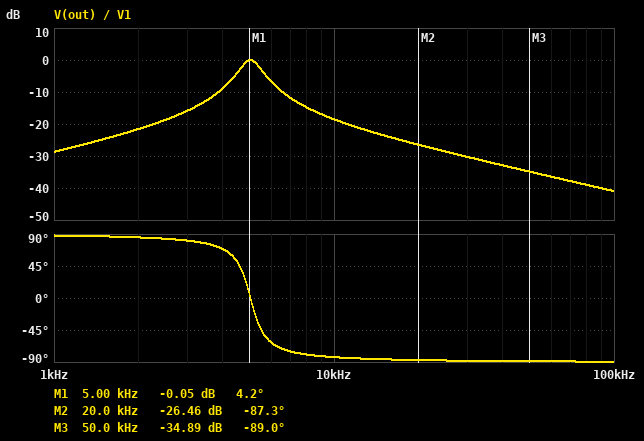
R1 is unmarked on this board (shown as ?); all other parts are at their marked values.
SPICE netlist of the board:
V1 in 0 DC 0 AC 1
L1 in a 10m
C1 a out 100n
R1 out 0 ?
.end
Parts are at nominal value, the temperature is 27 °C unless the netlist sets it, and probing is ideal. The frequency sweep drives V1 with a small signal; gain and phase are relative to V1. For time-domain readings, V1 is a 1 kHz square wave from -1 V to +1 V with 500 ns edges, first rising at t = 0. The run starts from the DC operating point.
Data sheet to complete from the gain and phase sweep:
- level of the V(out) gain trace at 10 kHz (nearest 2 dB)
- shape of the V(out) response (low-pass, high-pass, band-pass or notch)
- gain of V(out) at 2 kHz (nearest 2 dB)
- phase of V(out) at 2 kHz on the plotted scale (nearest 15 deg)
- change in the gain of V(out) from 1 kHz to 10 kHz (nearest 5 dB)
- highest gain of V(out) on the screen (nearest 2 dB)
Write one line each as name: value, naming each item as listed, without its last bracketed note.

level of the V(out) gain trace at 10 kHz: -18 dB
shape of the V(out) response: band-pass
gain of V(out) at 2 kHz: -22 dB
phase of V(out) at 2 kHz on the plotted scale: 90 deg
change in the gain of V(out) from 1 kHz to 10 kHz: 10 dB
highest gain of V(out) on the screen: 0 dB
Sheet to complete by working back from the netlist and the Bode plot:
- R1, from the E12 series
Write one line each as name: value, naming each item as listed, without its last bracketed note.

R1, from the E12 series: 56 Ω
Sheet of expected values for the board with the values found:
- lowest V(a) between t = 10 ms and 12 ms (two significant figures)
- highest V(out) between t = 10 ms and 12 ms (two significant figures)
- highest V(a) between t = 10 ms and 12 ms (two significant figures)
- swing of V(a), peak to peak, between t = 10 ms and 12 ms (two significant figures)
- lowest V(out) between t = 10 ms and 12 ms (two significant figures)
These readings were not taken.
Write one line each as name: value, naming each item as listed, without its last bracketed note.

lowest V(a) between t = 10 ms and 12 ms: -3.0 V
highest V(out) between t = 10 ms and 12 ms: 410 mV
highest V(a) between t = 10 ms and 12 ms: 3.0 V
swing of V(a), peak to peak, between t = 10 ms and 12 ms: 6.1 V
lowest V(out) between t = 10 ms and 12 ms: -410 mV
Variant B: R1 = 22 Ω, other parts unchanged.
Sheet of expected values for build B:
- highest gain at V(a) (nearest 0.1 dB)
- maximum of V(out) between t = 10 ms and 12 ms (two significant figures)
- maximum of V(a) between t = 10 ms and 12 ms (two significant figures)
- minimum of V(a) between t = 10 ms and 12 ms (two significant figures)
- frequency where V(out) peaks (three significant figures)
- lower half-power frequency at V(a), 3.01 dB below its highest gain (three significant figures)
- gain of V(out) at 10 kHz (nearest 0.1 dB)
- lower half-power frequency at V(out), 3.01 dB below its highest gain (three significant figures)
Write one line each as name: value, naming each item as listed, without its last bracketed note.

highest gain at V(a): 23.2 dB
maximum of V(out) between t = 10 ms and 12 ms: 310 mV
maximum of V(a) between t = 10 ms and 12 ms: 5.2 V
minimum of V(a) between t = 10 ms and 12 ms: -5.2 V
frequency where V(out) peaks: 5.03 kHz
lower half-power frequency at V(a), 3.01 dB below its highest gain: 4.85 kHz
gain of V(out) at 10 kHz: -26.6 dB
lower half-power frequency at V(out), 3.01 dB below its highest gain: 4.86 kHz
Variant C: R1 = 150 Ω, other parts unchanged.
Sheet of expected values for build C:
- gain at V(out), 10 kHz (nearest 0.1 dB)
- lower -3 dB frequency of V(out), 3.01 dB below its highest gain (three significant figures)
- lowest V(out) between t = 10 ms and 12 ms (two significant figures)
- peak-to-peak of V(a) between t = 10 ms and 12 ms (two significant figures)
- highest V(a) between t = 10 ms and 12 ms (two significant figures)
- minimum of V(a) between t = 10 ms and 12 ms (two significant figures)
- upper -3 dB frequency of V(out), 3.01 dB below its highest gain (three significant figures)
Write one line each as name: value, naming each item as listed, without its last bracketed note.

gain at V(out), 10 kHz: -10.3 dB
lower -3 dB frequency of V(out), 3.01 dB below its highest gain: 3.98 kHz
lowest V(out) between t = 10 ms and 12 ms: -700 mV
peak-to-peak of V(a) between t = 10 ms and 12 ms: 4.1 V
highest V(a) between t = 10 ms and 12 ms: 2.1 V
minimum of V(a) between t = 10 ms and 12 ms: -2.1 V
upper -3 dB frequency of V(out), 3.01 dB below its highest gain: 6.37 kHz
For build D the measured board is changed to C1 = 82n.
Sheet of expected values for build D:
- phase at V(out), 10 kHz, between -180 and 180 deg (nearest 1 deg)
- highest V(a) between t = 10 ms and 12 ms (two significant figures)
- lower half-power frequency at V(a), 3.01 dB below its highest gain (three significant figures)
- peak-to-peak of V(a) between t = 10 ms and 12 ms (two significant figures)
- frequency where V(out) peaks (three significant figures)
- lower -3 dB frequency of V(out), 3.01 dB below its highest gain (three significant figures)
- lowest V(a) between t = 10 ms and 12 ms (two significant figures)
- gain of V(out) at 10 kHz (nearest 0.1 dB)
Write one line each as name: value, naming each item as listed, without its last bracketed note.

phase at V(out), 10 kHz, between -180 and 180 deg: -83 deg
highest V(a) between t = 10 ms and 12 ms: 2.5 V
lower half-power frequency at V(a), 3.01 dB below its highest gain: 5.06 kHz
peak-to-peak of V(a) between t = 10 ms and 12 ms: 5.0 V
frequency where V(out) peaks: 5.56 kHz
lower -3 dB frequency of V(out), 3.01 dB below its highest gain: 5.13 kHz
lowest V(a) between t = 10 ms and 12 ms: -2.5 V
gain of V(out) at 10 kHz: -17.9 dB
